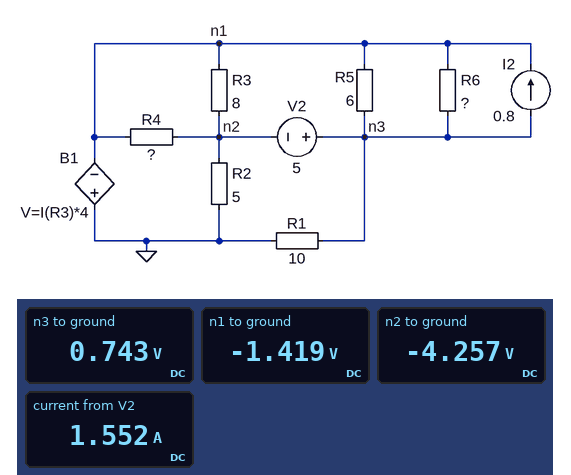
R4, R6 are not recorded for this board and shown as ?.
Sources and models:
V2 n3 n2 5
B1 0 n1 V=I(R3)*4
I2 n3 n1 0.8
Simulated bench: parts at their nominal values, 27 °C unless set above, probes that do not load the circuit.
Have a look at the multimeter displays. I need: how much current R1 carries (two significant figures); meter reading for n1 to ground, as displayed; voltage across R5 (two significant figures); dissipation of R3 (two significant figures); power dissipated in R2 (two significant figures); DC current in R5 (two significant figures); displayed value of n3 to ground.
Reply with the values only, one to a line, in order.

74 mA
-1.419 V
2.2 V
1.0 W
3.6 W
360 mA
0.743 V
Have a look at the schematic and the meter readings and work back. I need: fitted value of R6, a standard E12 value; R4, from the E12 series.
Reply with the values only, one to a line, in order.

6.8 Ω
8.2 Ω
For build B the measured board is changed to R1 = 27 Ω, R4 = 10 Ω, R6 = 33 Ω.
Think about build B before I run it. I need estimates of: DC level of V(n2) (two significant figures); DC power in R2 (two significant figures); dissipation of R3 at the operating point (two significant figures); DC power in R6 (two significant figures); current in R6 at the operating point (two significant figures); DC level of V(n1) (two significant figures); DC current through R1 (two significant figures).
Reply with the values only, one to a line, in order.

-3.8 V
2.9 W
800 mW
180 mW
75 mA
-1.3 V
44 mA
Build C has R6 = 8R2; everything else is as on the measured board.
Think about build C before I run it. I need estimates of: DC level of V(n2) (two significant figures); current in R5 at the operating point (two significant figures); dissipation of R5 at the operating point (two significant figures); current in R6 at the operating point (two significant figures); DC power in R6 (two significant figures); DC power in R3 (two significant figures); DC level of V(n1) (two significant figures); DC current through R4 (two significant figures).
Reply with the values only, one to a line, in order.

-4.2 V
370 mA
820 mW
270 mA
600 mW
970 mW
-1.4 V
340 mA
